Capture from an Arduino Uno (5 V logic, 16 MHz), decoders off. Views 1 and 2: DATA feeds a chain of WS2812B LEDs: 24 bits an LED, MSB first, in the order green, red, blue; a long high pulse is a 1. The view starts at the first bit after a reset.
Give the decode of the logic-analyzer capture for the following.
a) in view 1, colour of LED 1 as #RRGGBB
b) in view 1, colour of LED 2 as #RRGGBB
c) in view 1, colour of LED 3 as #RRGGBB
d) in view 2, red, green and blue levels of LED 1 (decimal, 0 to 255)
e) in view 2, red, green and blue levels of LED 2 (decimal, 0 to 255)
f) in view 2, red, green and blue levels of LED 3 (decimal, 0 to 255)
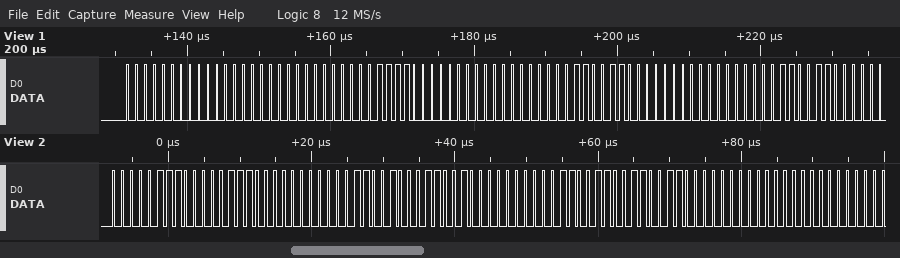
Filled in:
#000000
#000F00
#003300
7, 7, 0
25, 25, 0
51, 51, 0
